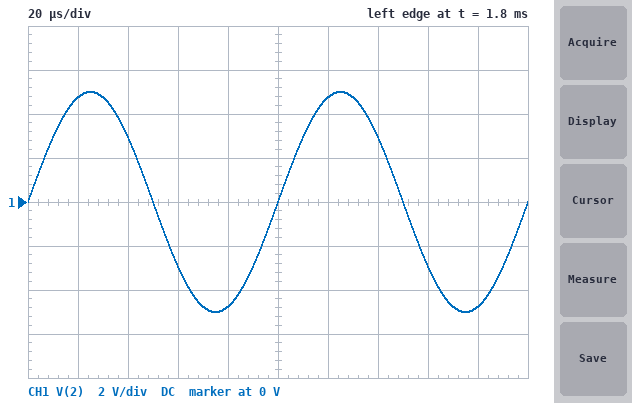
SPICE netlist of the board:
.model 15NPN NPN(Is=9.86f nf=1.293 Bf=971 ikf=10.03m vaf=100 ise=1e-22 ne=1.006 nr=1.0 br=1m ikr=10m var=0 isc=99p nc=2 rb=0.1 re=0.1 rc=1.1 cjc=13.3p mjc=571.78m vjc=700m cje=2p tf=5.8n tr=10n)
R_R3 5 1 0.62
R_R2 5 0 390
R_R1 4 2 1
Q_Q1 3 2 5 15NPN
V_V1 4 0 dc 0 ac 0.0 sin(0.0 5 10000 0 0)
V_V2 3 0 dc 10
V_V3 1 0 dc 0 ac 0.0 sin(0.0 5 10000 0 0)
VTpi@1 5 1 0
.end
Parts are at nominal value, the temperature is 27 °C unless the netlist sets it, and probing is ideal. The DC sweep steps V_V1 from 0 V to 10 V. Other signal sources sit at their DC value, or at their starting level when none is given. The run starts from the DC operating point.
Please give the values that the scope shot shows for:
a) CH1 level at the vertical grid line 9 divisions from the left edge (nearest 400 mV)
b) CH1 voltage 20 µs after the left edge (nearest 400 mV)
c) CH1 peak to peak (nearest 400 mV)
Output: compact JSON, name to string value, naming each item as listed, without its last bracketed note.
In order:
{"CH1 level at the vertical grid line 9 divisions from the left edge": "-4.8 V", "CH1 voltage 20 µs after the left edge": "4.8 V", "CH1 peak to peak": "10.0 V"}
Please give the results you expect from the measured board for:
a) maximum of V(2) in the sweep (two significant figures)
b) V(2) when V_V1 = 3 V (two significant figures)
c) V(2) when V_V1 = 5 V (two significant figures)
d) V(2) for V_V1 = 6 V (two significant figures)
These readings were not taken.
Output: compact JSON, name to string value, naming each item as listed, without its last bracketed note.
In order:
{"maximum of V(2) in the sweep": "3.3 V", "V(2) when V_V1 = 3 V": "1.8 V", "V(2) when V_V1 = 5 V": "2.3 V", "V(2) for V_V1 = 6 V": "2.5 V"}
